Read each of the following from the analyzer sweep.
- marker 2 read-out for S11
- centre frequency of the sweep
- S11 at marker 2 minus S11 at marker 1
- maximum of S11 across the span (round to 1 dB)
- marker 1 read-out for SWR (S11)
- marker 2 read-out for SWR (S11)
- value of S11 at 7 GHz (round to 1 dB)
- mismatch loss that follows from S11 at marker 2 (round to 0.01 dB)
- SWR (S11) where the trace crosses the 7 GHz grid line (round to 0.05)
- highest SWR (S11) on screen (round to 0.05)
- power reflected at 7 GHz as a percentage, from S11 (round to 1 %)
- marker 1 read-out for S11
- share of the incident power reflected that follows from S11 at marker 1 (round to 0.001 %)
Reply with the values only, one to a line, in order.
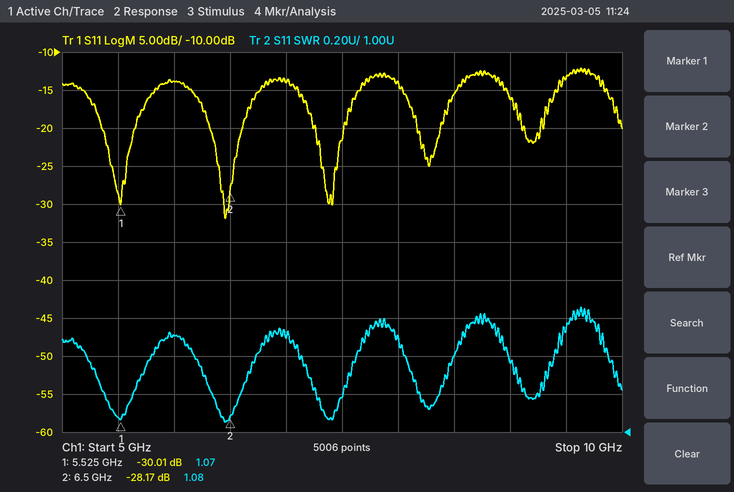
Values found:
-28.17 dB
7.5 GHz
1.84 dB
-12 dB
1.07
1.08
-14 dB
0.01 dB
1.50
1.65
4 %
-30.01 dB
0.100 %
